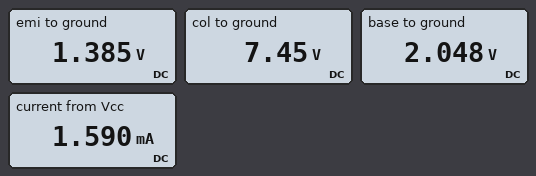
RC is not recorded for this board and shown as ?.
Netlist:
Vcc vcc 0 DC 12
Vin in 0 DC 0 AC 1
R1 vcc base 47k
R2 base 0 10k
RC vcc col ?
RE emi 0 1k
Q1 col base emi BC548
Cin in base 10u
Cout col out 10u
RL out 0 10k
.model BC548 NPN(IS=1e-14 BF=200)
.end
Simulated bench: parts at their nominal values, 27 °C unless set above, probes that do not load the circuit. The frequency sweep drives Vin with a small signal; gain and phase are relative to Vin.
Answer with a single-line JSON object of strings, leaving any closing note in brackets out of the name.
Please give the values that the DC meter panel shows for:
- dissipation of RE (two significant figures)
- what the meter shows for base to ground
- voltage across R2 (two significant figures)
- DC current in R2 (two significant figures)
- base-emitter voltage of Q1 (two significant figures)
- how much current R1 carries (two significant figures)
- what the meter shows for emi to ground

{"dissipation of RE": "1.9 mW", "what the meter shows for base to ground": "2.048 V", "voltage across R2": "2.0 V", "DC current in R2": "200 µA", "base-emitter voltage of Q1": "660 mV", "how much current R1 carries": "210 µA", "what the meter shows for emi to ground": "1.385 V"}
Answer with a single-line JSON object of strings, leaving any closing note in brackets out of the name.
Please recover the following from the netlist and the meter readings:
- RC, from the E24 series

{"RC, from the E24 series": "3.3 kΩ"}
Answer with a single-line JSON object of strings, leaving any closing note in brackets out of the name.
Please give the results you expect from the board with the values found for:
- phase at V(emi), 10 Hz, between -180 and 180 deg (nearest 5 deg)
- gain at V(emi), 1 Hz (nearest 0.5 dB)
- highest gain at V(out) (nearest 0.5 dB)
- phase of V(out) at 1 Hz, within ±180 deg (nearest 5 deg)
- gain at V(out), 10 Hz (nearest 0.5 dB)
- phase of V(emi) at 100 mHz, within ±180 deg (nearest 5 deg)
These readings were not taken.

{"phase at V(emi), 10 Hz, between -180 and 180 deg": "10 deg", "gain at V(emi), 1 Hz": "-7.0 dB", "highest gain at V(out)": "7.5 dB", "phase of V(out) at 1 Hz, within ±180 deg": "-65 deg", "gain at V(out), 10 Hz": "7.5 dB", "phase of V(emi) at 100 mHz, within ±180 deg": "85 deg"}
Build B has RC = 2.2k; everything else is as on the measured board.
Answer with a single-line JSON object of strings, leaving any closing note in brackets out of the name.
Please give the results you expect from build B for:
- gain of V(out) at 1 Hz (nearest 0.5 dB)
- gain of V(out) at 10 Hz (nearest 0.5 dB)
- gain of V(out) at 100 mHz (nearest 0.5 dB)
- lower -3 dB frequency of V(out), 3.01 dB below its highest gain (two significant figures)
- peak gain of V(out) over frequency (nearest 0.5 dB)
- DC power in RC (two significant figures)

{"gain of V(out) at 1 Hz": "-6.5 dB", "gain of V(out) at 10 Hz": "4.5 dB", "gain of V(out) at 100 mHz": "-43.5 dB", "lower -3 dB frequency of V(out), 3.01 dB below its highest gain": "2.6 Hz", "peak gain of V(out) over frequency": "5.0 dB", "DC power in RC": "4.2 mW"}
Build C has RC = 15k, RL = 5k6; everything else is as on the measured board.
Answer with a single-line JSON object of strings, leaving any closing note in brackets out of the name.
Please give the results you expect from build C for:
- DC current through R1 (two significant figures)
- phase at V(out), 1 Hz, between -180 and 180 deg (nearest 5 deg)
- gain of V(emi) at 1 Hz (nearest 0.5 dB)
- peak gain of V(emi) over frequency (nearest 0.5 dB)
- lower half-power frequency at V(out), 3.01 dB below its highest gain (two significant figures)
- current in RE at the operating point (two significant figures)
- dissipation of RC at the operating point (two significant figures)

{"DC current through R1": "220 µA", "phase at V(out), 1 Hz, between -180 and 180 deg": "155 deg", "gain of V(emi) at 1 Hz": "-25.5 dB", "peak gain of V(emi) over frequency": "-0.5 dB", "lower half-power frequency at V(out), 3.01 dB below its highest gain": "20 Hz", "current in RE at the operating point": "820 µA", "dissipation of RC at the operating point": "8.2 mW"}
